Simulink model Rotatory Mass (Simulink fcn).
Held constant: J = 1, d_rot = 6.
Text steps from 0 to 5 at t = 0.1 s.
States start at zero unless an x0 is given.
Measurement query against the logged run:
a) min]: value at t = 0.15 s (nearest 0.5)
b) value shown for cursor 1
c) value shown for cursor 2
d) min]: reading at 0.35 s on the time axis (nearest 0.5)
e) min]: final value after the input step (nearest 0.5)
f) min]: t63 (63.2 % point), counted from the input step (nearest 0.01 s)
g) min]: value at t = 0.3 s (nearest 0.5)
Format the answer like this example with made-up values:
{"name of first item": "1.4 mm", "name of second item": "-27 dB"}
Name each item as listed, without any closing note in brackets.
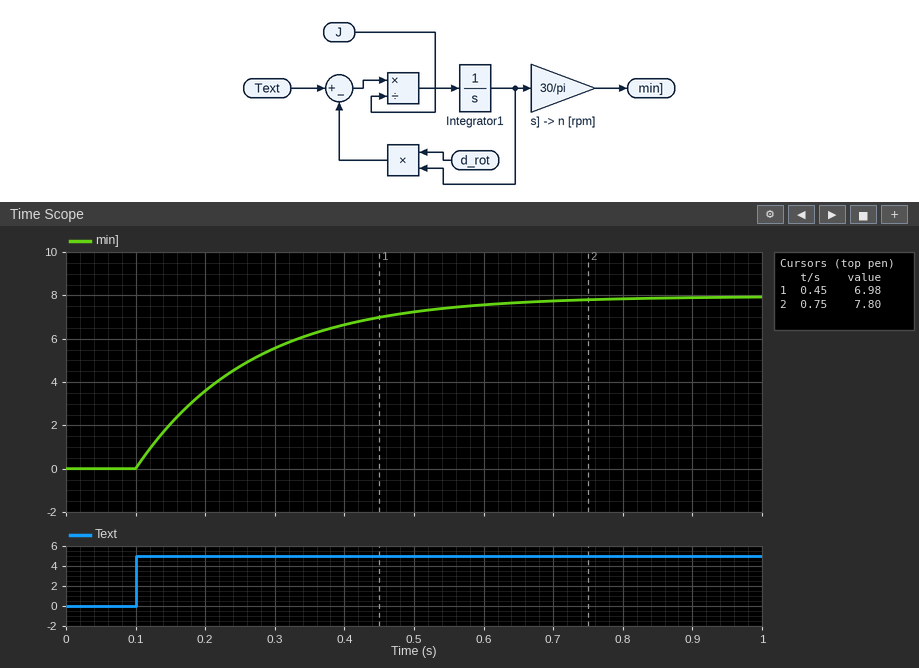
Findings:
{"min]: value at t = 0.15 s": "2.0", "value shown for cursor 1": "6.98", "value shown for cursor 2": "7.80", "min]: reading at 0.35 s on the time axis": "6.0", "min]: final value after the input step": "8.0", "min]: t63 (63.2 % point), counted from the input step": "0.17 s", "min]: value at t = 0.3 s": "5.5"}
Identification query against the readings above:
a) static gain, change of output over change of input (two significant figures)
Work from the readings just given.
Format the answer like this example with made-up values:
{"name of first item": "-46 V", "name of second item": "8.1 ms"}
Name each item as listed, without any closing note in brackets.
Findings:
{"static gain, change of output over change of input": "1.6"}
